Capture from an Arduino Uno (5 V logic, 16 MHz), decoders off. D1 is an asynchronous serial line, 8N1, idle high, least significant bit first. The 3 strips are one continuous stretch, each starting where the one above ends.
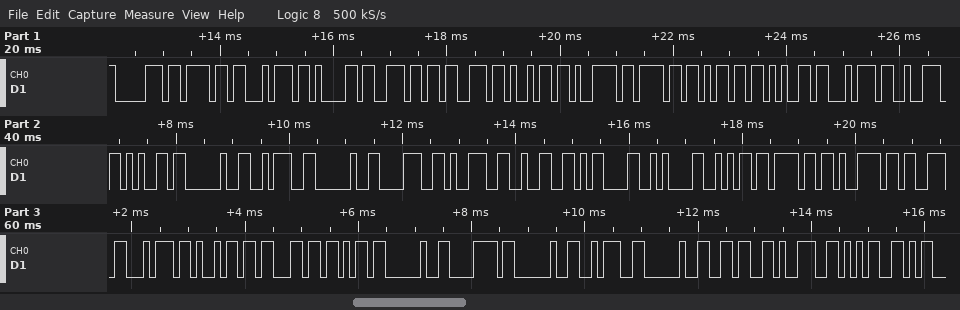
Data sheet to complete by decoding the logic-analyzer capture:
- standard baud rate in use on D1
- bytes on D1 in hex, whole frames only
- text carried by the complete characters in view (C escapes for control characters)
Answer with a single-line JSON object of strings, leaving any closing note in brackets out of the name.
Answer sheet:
{"standard baud rate in use on D1": "9600 baud", "bytes on D1 in hex, whole frames only": "70 6F 74 61 6E 73 69 79 6F 6D 65 74 72 65 20 3A 20 38 39 32 0D 0A 6A 6F 79 73 74 69 63 6B 20 78 20 3A 20 36 39 35", "text carried by the complete characters in view": "\"potansiyometre : 892\\r\\njoystick x : 695\""}
